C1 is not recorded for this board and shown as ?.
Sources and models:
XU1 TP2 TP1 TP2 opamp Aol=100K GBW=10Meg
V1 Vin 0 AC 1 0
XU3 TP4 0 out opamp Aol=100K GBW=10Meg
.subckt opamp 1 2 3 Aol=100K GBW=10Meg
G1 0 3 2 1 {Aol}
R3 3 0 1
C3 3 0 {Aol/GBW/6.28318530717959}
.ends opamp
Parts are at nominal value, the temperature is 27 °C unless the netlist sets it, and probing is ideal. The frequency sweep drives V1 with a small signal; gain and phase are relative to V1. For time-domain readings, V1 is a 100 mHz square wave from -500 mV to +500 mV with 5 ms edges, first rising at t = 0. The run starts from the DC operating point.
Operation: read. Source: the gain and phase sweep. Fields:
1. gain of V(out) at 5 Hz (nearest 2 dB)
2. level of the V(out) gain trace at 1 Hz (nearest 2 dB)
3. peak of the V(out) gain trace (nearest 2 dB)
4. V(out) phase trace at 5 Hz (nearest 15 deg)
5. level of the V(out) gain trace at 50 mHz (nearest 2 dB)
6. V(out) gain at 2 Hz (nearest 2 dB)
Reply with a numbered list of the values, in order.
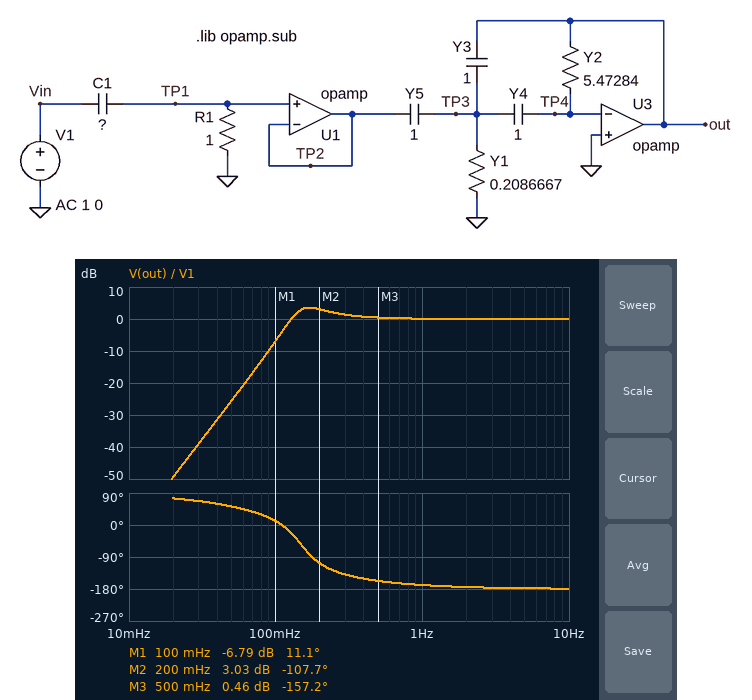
1. 0 dB
2. 0 dB
3. 4 dB
4. -180 deg
5. -26 dB
6. 0 dB
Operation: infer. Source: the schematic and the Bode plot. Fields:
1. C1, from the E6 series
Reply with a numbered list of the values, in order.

1. 1.5 F
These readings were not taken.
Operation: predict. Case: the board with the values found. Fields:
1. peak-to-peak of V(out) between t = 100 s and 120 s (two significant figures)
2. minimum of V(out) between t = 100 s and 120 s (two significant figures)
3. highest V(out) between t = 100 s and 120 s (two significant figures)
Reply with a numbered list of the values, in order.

1. 1.5 V
2. -760 mV
3. 760 mV
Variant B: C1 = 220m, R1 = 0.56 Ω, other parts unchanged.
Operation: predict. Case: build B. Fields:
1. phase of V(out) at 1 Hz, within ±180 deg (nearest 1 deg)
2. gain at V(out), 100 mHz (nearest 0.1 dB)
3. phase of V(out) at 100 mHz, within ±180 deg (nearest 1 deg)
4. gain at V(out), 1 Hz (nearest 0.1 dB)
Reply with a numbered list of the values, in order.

1. -123 deg
2. -25.8 dB
3. 50 deg
4. -4.1 dB
